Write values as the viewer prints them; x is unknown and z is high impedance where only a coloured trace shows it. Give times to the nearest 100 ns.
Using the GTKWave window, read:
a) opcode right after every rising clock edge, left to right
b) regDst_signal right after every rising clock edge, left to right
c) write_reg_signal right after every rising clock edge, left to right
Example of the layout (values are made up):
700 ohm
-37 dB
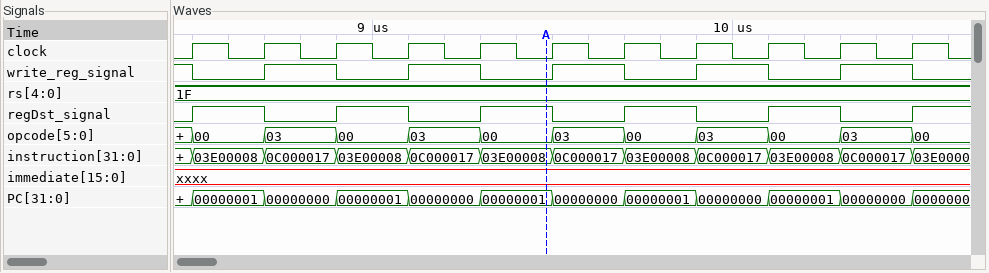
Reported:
00, 03, 00, 03, 00, 03, 00, 03, 00, 03, 00
1 0 1 0 1 0 1 0 1 0 1
0 1 0 1 0 1 0 1 0 1 0
